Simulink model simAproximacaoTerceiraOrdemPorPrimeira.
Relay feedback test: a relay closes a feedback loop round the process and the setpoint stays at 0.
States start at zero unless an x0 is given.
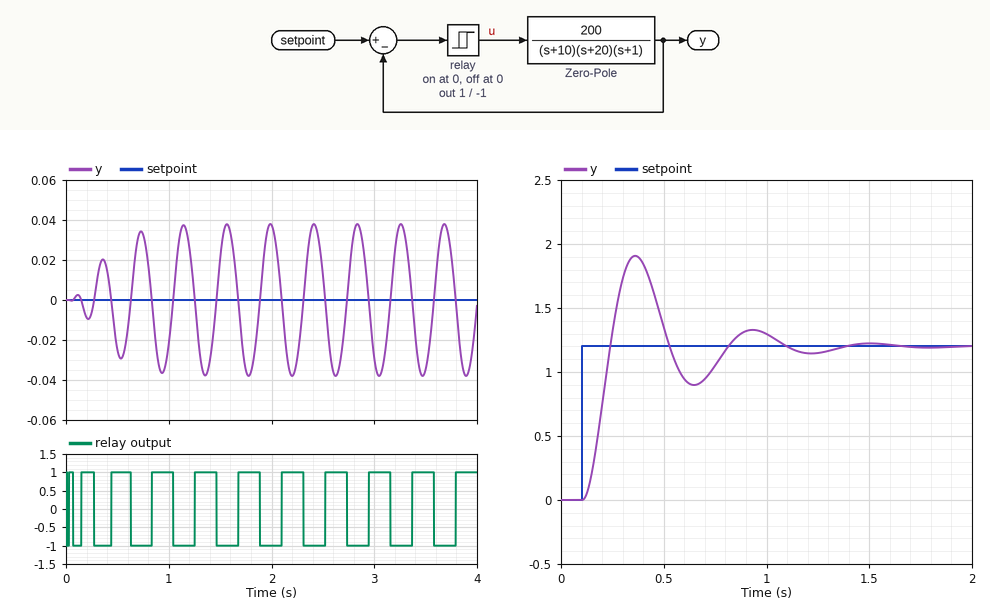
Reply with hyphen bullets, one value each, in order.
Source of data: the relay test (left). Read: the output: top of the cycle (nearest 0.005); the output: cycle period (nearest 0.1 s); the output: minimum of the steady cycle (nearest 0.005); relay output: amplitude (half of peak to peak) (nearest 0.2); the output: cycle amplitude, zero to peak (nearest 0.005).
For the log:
- 0.040
- 0.4 s
- -0.040
- 1.0
- 0.040
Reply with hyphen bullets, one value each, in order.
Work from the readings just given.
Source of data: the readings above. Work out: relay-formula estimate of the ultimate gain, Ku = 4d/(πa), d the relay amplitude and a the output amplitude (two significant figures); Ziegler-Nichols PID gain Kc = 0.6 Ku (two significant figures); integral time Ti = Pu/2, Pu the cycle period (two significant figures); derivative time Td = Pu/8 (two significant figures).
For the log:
- 32
- 19
- 0.20 s
- 0.050 s
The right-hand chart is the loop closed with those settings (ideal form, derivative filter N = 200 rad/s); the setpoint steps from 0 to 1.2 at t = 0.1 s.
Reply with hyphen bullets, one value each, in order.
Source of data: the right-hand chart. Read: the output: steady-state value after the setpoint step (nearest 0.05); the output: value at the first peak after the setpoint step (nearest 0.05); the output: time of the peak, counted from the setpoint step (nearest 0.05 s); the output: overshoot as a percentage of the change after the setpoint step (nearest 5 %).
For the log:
- 1.20
- 1.90
- 0.25 s
- 60 %
